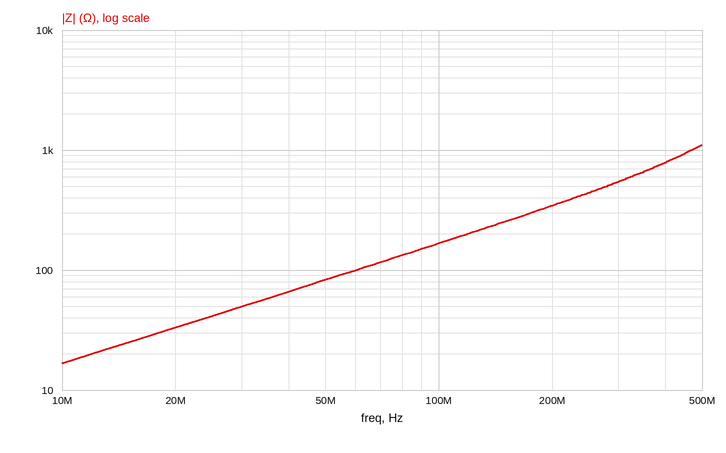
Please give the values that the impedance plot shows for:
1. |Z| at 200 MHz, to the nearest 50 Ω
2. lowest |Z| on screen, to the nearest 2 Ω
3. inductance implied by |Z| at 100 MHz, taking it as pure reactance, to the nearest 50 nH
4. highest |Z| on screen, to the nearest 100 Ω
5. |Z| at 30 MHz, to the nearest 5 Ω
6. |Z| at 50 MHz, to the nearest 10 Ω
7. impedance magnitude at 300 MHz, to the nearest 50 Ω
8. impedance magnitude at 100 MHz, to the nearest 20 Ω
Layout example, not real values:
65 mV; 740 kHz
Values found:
350 Ω; 16 Ω; 250 nH; 1.1 kΩ; 50 Ω; 80 Ω; 550 Ω; 160 Ω
